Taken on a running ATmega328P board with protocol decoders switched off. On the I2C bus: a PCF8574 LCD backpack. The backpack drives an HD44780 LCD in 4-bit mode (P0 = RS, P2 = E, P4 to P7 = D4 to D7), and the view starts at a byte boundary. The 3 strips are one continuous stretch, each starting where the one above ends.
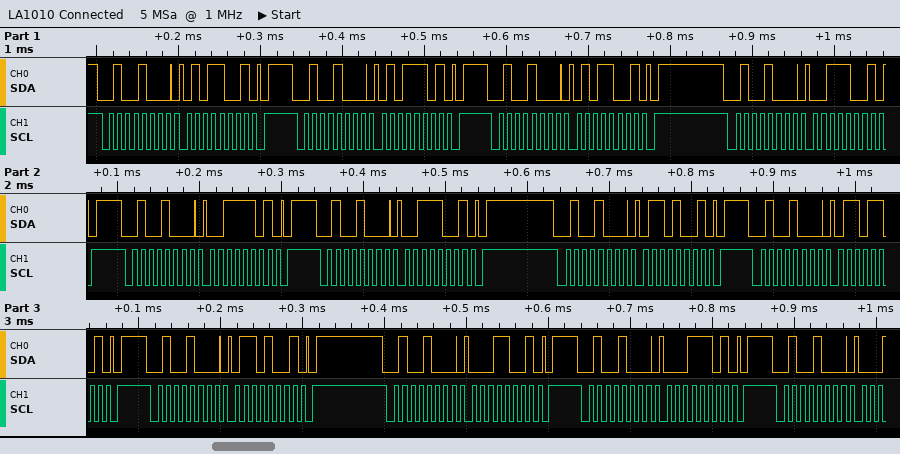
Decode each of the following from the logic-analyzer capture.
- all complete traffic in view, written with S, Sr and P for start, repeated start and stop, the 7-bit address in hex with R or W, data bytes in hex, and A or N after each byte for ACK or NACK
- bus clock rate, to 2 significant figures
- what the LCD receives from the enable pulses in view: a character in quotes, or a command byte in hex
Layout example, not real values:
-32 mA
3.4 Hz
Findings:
S 24W A 59 A P S 24W A 5D A P S 24W A 59 A P S 24W A 39 A P S 24W A 3D A P S 24W A 39 A P S 24W A 69 A P S 24W A 6D A P S 24W A 69 A P S 24W A 19 A P S 24W A 1D A P S 24W A
100 kHz
'S'
